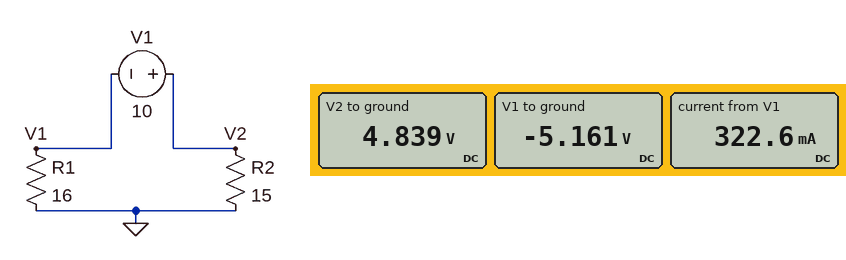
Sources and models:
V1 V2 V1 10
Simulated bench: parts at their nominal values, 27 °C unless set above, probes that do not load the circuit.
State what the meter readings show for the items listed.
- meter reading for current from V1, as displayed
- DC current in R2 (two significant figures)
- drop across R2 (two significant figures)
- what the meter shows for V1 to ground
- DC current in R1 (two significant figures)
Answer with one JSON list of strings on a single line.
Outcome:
["322.6 mA", "320 mA", "4.8 V", "-5.161 V", "320 mA"]
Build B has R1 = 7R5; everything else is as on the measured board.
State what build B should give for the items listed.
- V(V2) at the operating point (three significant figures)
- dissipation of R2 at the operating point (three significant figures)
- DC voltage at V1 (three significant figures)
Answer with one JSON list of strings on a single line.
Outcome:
["6.67 V", "2.96 W", "-3.33 V"]
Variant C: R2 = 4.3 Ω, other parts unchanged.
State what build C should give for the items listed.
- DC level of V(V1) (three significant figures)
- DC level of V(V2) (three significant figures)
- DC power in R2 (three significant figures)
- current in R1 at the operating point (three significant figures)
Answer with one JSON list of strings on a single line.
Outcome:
["-7.88 V", "2.12 V", "1.04 W", "493 mA"]
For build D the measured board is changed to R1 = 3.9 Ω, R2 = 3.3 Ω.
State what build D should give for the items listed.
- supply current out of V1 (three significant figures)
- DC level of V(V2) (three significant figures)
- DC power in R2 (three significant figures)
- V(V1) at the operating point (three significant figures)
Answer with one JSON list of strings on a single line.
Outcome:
["1.39 A", "4.58 V", "6.37 W", "-5.42 V"]
